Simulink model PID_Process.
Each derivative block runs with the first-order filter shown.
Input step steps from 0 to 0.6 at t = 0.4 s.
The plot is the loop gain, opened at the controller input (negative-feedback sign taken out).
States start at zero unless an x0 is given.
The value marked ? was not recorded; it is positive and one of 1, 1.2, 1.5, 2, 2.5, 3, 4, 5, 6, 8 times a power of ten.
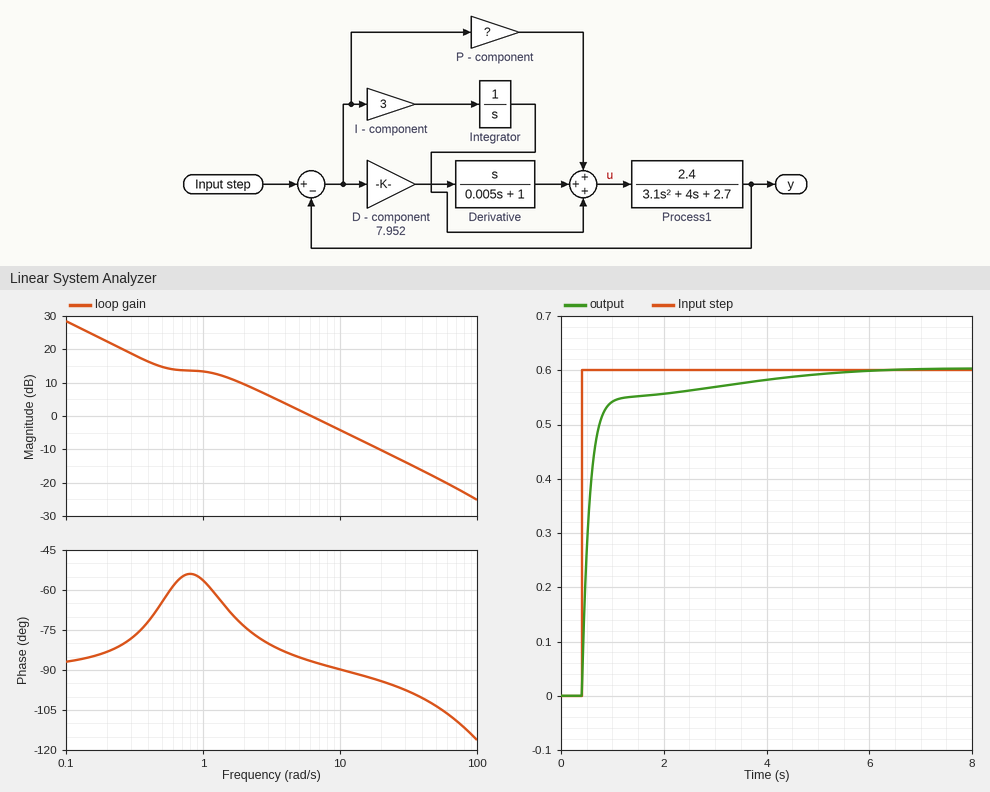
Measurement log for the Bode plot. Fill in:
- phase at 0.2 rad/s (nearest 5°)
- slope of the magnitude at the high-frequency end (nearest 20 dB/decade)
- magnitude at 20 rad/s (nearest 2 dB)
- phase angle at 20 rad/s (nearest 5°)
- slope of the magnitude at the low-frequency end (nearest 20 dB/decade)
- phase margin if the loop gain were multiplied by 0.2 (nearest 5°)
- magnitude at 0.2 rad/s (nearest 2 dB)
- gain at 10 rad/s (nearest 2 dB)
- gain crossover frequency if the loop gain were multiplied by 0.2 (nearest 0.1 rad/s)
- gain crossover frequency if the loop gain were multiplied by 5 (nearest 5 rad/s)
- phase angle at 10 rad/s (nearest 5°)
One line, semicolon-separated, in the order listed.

-85°; -20 dB/decade; -10 dB; -95°; -20 dB/decade; 120°; 22 dB; -4 dB; 0.6 rad/s; 30 rad/s; -90°
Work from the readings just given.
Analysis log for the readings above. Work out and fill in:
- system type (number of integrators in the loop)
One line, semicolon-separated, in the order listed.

1
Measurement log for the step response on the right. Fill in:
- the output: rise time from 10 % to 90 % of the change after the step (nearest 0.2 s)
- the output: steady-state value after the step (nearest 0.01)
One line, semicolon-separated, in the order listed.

0.6 s; 0.60
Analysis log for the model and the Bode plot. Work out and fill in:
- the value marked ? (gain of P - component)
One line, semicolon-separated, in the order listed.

6
